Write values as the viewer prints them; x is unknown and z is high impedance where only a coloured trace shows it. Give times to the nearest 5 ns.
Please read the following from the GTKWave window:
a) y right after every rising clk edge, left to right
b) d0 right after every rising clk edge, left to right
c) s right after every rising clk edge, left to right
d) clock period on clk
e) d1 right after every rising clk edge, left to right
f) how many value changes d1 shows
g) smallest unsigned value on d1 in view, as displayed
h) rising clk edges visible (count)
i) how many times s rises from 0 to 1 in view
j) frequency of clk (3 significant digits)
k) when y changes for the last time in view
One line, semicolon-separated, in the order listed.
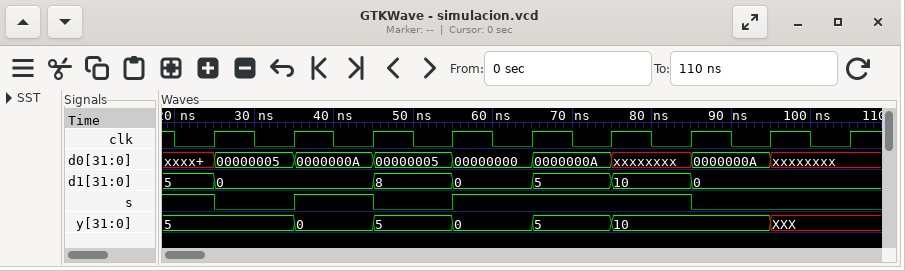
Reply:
5, 0, 5, 0, 5, 10, 10, XXX, XXX; 00000005, 0000000A, 00000005, 00000000, 0000000A, xxxxxxxx, 0000000A, xxxxxxxx, xxxxxxxx; 0 1 0 1 1 1 0 0 0; 10 ns; 0, 0, 8, 0, 5, 10, 0, 0, 0; 6; 0; 9; 2; 100 MHz; 95 ns
